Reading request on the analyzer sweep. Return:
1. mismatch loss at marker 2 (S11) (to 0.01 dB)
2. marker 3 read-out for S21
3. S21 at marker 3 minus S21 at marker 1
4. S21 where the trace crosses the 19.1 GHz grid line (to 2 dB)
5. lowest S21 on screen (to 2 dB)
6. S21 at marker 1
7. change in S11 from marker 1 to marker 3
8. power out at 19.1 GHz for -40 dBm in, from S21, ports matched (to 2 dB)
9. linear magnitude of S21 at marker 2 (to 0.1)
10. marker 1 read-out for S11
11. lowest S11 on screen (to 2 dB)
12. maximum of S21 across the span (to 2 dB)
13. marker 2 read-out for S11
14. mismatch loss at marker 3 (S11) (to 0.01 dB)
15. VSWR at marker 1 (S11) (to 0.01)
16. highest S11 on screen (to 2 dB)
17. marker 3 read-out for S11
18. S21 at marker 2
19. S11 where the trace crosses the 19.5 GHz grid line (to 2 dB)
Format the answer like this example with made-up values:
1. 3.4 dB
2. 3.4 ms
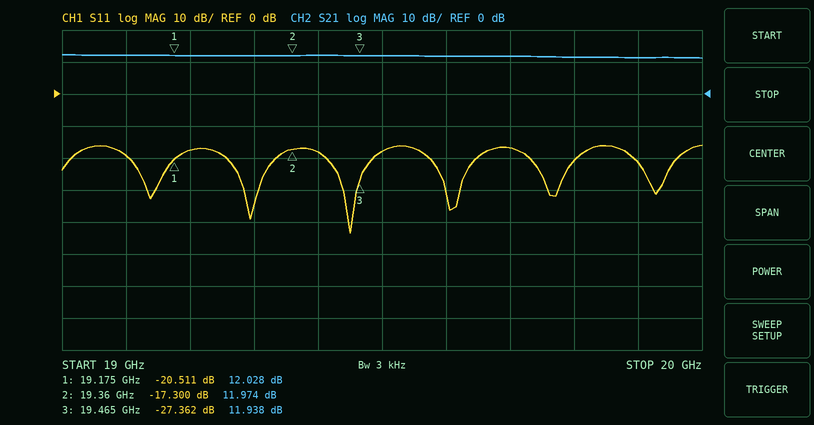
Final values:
1. 0.08 dB
2. 11.938 dB
3. -0.090 dB
4. 12 dB
5. 12 dB
6. 12.028 dB
7. -6.851 dB
8. -28 dBm
9. 4.0
10. -20.511 dB
11. -44 dB
12. 12 dB
13. -17.300 dB
14. 0.01 dB
15. 1.21
16. -16 dB
17. -27.362 dB
18. 11.974 dB
19. -18 dB
